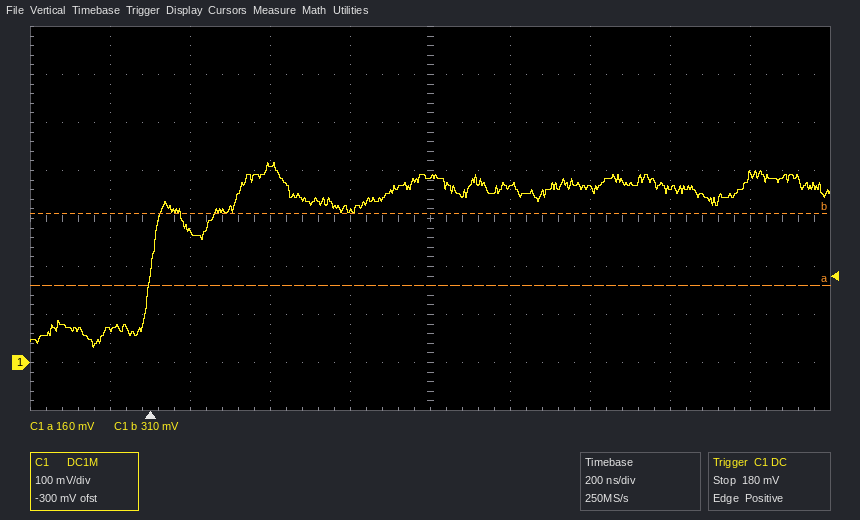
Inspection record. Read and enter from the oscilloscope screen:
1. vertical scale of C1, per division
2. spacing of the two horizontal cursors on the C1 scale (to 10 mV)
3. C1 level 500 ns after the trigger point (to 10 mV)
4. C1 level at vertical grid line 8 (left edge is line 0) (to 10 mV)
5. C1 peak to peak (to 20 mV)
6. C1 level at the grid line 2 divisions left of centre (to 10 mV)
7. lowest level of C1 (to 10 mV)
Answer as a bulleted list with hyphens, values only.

- 100 mV
- 150 mV
- 320 mV
- 360 mV
- 380 mV
- 410 mV
- 30 mV
